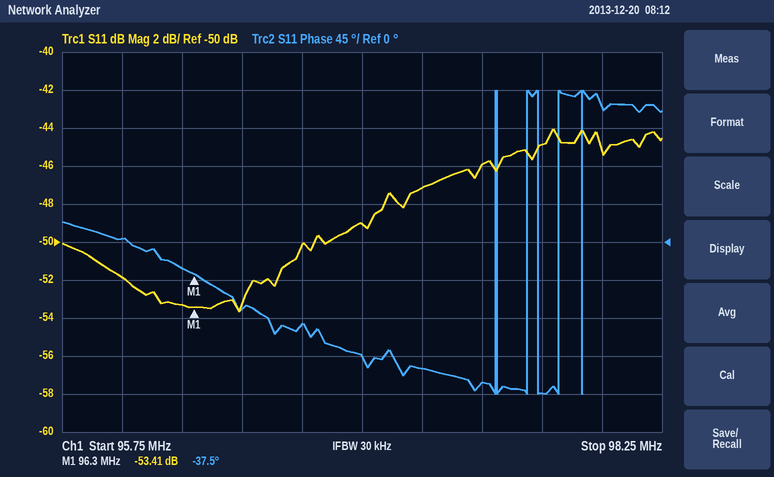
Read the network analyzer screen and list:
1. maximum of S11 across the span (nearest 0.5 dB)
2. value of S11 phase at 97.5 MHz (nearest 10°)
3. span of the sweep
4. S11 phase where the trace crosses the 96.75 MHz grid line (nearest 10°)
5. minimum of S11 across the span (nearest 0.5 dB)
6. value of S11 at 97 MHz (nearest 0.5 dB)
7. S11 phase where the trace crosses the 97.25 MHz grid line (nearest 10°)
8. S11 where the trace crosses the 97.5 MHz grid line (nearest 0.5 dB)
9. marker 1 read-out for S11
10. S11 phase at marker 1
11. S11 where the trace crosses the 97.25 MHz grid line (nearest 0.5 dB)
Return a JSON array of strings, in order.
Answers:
["-44.0 dB", "-170°", "2.5 MHz", "-100°", "-53.5 dB", "-49.0 dB", "-150°", "-46.0 dB", "-53.41 dB", "-37.5°", "-47.0 dB"]
